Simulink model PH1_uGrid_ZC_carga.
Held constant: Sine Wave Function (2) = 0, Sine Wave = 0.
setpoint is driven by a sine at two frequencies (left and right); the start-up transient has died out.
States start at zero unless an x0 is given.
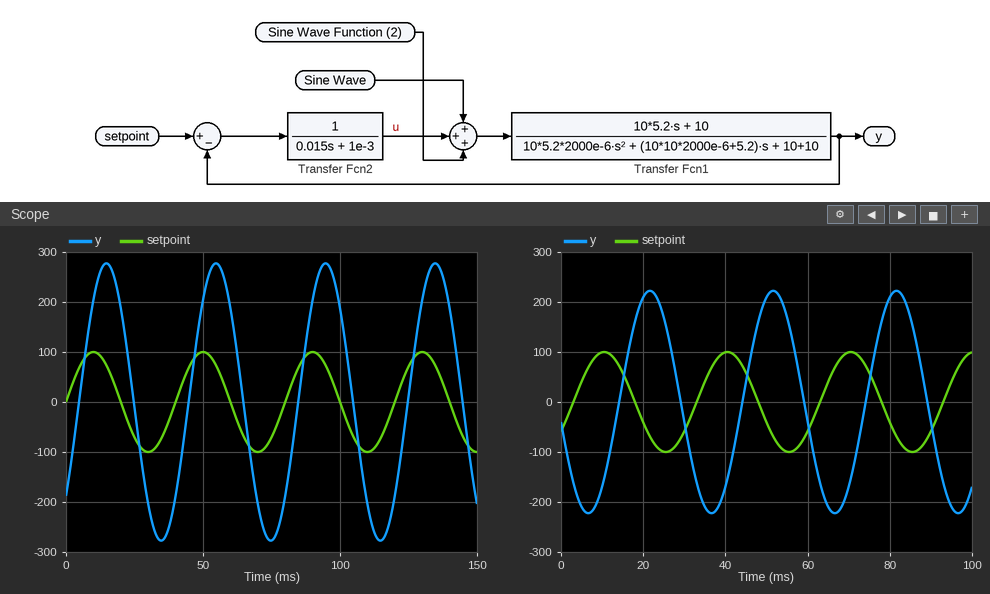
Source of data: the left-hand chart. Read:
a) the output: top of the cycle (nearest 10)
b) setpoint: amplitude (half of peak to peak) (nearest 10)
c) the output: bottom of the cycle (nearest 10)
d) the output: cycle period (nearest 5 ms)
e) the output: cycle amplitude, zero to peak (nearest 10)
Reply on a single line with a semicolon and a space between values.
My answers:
280; 100; -280; 40 ms; 280
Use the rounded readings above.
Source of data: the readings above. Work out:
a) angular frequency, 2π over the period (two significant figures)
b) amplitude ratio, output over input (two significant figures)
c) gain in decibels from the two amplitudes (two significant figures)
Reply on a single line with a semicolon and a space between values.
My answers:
0.16 rad/ms; 2.8; 8.9 dB
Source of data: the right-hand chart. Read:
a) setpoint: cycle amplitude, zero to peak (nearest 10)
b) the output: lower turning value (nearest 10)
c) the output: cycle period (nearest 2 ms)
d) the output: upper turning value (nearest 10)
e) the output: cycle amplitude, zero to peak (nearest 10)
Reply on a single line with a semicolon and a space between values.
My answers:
100; -220; 30 ms; 220; 220
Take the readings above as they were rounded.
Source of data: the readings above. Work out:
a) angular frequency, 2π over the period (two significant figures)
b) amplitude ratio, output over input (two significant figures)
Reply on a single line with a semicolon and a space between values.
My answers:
0.21 rad/ms; 2.2
